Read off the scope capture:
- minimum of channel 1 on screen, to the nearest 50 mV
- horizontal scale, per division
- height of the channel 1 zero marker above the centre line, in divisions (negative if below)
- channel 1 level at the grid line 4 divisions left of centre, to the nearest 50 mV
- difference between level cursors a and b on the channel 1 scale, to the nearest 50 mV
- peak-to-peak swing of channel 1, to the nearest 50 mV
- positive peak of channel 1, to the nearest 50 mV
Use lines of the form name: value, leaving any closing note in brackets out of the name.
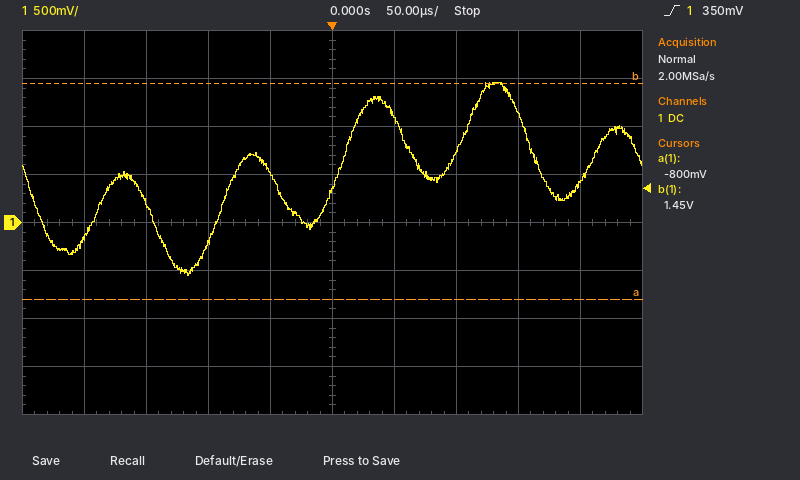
minimum of channel 1 on screen, to the nearest 50 mV: -550 mV
horizontal scale, per division: 50 µs
height of the channel 1 zero marker above the centre line, in divisions: 0.0 div
channel 1 level at the grid line 4 divisions left of centre, to the nearest 50 mV: -150 mV
difference between level cursors a and b on the channel 1 scale, to the nearest 50 mV: 2.25 V
peak-to-peak swing of channel 1, to the nearest 50 mV: 2.00 V
positive peak of channel 1, to the nearest 50 mV: 1.45 V
